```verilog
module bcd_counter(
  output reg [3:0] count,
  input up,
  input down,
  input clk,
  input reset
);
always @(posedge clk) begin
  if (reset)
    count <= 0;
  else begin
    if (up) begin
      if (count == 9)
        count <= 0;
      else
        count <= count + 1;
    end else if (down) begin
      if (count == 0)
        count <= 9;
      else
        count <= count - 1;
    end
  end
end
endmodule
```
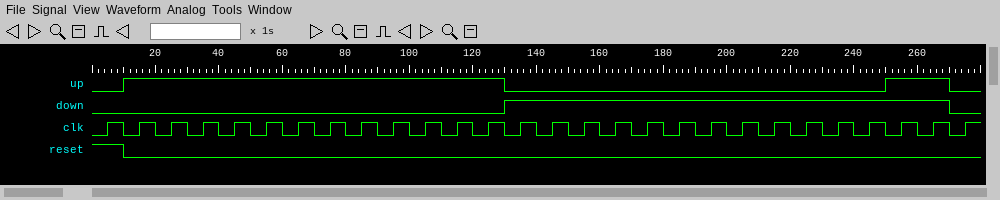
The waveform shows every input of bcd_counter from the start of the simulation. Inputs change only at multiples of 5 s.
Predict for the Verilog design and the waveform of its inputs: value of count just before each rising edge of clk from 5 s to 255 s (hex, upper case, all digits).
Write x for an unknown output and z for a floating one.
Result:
x, 0, 1, 2, 3, 4, 5, 6, 7, 8, 9, 0, 1, 2, 1, 0, 9, 8, 7, 6, 5, 4, 3, 2, 1, 0
